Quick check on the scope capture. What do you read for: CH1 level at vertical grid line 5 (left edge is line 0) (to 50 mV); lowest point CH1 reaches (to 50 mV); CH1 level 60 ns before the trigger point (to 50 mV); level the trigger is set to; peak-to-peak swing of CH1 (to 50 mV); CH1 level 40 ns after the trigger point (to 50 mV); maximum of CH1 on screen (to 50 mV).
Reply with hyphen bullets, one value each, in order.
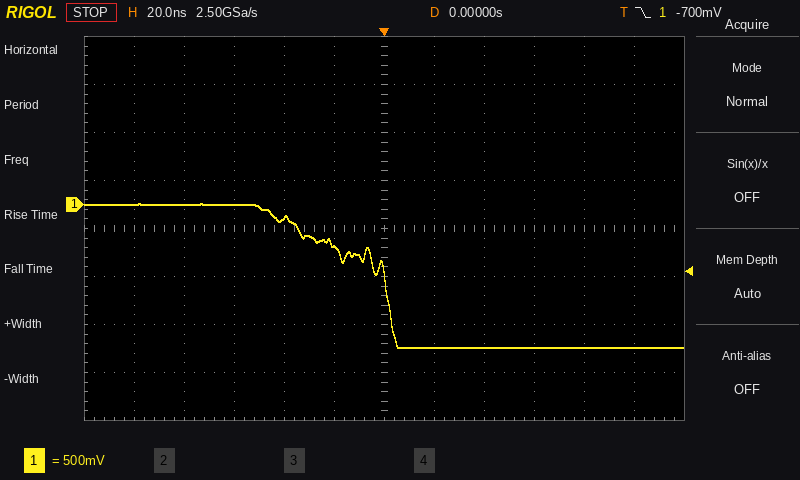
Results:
- -450 mV
- -1.50 V
- 0 mV
- -700 mV
- 1.50 V
- -1.50 V
- 0 mV
